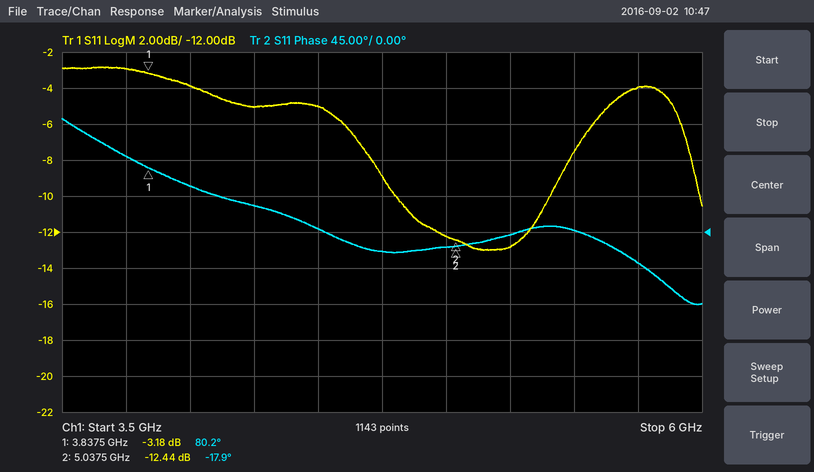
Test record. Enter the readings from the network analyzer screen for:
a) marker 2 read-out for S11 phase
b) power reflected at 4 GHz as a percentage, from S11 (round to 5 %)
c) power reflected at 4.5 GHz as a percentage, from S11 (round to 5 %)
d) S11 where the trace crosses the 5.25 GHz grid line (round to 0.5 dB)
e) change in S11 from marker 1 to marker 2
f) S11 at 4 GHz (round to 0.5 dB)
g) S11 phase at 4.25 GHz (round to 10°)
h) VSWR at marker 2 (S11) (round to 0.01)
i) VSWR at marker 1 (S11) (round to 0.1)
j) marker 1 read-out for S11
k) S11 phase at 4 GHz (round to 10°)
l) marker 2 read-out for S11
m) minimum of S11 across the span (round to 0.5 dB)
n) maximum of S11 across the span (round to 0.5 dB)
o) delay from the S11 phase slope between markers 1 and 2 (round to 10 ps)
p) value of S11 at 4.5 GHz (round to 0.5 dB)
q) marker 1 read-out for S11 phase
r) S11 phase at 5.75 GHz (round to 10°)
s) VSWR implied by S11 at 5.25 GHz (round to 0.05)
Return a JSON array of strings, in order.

["-17.9°", "40 %", "30 %", "-13.0 dB", "-9.26 dB", "-4.0 dB", "30°", "1.63", "5.5", "-3.18 dB", "60°", "-12.44 dB", "-13.0 dB", "-3.0 dB", "230 ps", "-5.0 dB", "80.2°", "-40°", "1.60"]
